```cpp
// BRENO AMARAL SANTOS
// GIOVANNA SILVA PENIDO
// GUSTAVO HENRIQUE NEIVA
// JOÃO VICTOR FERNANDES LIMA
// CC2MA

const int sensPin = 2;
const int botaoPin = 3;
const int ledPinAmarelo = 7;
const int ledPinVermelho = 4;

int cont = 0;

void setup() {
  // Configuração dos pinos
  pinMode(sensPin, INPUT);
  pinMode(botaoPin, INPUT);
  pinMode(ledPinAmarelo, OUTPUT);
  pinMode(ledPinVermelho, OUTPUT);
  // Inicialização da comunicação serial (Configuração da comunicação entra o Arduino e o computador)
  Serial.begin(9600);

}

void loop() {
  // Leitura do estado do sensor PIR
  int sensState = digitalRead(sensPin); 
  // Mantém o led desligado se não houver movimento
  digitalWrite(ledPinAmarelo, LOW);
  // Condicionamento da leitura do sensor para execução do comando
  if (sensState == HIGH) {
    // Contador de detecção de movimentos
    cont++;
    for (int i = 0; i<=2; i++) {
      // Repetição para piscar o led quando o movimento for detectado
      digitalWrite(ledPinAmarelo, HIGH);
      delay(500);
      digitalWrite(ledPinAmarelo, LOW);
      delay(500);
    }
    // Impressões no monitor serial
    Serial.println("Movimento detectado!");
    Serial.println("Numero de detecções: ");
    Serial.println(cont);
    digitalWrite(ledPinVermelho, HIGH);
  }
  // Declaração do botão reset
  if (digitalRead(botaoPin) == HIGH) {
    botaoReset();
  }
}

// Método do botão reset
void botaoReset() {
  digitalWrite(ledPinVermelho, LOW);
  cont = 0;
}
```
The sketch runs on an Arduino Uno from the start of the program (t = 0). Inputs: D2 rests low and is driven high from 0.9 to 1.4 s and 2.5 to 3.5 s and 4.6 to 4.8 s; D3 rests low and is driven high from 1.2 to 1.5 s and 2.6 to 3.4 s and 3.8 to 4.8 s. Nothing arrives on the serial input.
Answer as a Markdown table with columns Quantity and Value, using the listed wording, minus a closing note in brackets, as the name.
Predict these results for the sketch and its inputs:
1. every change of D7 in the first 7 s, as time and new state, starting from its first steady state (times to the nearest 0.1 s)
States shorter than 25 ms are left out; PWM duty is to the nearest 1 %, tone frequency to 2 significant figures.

| Quantity | Value |
|---|---|
| every change of D7 in the first 7 s, as time and new state, starting from its first steady state | 0 s low; 0.9 s high; 1.4 s low; 1.9 s high; 2.4 s low; 2.9 s high; 3.4 s low; 4.6 s high; 5.1 s low; 5.6 s high; 6.1 s low; 6.6 s high |
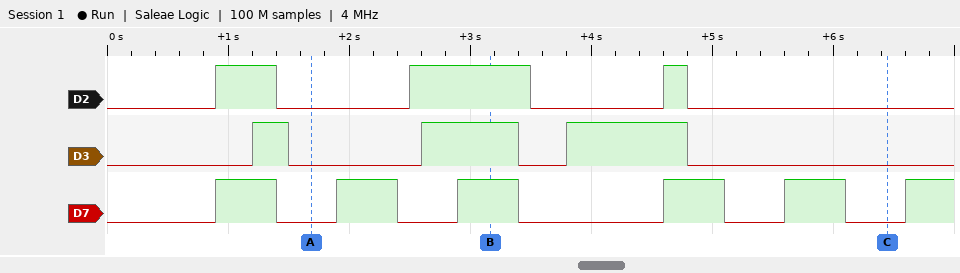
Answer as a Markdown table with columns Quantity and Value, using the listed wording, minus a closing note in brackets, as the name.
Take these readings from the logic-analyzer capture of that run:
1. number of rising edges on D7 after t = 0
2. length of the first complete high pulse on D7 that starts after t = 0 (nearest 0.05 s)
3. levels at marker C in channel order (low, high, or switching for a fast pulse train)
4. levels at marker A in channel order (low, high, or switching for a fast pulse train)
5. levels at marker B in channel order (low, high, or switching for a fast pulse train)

| Quantity | Value |
|---|---|
| number of rising edges on D7 after t = 0 | 6 |
| length of the first complete high pulse on D7 that starts after t = 0 | 0.50 s |
| levels at marker C in channel order | D2 low, D3 low, D7 low |
| levels at marker A in channel order | D2 low, D3 low, D7 low |
| levels at marker B in channel order | D2 high, D3 high, D7 high |
